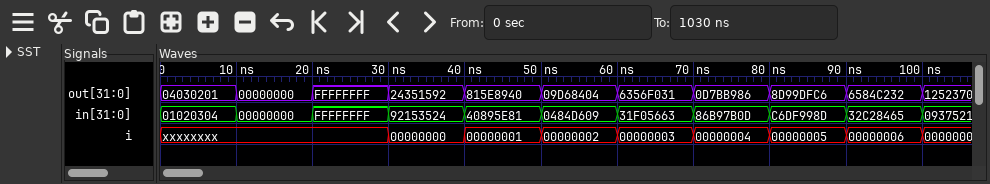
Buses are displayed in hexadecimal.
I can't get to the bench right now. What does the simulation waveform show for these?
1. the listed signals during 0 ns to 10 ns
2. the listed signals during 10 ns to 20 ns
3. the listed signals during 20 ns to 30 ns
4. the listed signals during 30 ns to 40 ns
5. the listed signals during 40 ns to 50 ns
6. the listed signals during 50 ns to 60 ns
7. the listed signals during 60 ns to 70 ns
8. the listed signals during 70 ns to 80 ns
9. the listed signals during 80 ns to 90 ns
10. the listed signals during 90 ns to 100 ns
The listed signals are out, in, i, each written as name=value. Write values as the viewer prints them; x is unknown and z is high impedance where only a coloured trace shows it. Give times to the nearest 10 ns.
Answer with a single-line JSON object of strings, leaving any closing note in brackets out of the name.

{"the listed signals during 0 ns to 10 ns": "out=04030201, in=01020304, i=xxxxxxxx", "the listed signals during 10 ns to 20 ns": "out=00000000, in=00000000, i=xxxxxxxx", "the listed signals during 20 ns to 30 ns": "out=FFFFFFFF, in=FFFFFFFF, i=xxxxxxxx", "the listed signals during 30 ns to 40 ns": "out=24351592, in=92153524, i=00000000", "the listed signals during 40 ns to 50 ns": "out=815E8940, in=40895E81, i=00000001", "the listed signals during 50 ns to 60 ns": "out=09D68404, in=0484D609, i=00000002", "the listed signals during 60 ns to 70 ns": "out=6356F031, in=31F05663, i=00000003", "the listed signals during 70 ns to 80 ns": "out=0D7BB986, in=86B97B0D, i=00000004", "the listed signals during 80 ns to 90 ns": "out=8D99DFC6, in=C6DF998D, i=00000005", "the listed signals during 90 ns to 100 ns": "out=6584C232, in=32C28465, i=00000006"}
